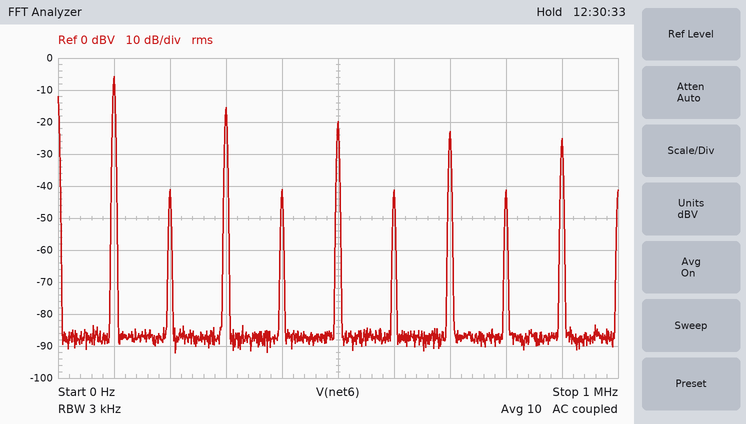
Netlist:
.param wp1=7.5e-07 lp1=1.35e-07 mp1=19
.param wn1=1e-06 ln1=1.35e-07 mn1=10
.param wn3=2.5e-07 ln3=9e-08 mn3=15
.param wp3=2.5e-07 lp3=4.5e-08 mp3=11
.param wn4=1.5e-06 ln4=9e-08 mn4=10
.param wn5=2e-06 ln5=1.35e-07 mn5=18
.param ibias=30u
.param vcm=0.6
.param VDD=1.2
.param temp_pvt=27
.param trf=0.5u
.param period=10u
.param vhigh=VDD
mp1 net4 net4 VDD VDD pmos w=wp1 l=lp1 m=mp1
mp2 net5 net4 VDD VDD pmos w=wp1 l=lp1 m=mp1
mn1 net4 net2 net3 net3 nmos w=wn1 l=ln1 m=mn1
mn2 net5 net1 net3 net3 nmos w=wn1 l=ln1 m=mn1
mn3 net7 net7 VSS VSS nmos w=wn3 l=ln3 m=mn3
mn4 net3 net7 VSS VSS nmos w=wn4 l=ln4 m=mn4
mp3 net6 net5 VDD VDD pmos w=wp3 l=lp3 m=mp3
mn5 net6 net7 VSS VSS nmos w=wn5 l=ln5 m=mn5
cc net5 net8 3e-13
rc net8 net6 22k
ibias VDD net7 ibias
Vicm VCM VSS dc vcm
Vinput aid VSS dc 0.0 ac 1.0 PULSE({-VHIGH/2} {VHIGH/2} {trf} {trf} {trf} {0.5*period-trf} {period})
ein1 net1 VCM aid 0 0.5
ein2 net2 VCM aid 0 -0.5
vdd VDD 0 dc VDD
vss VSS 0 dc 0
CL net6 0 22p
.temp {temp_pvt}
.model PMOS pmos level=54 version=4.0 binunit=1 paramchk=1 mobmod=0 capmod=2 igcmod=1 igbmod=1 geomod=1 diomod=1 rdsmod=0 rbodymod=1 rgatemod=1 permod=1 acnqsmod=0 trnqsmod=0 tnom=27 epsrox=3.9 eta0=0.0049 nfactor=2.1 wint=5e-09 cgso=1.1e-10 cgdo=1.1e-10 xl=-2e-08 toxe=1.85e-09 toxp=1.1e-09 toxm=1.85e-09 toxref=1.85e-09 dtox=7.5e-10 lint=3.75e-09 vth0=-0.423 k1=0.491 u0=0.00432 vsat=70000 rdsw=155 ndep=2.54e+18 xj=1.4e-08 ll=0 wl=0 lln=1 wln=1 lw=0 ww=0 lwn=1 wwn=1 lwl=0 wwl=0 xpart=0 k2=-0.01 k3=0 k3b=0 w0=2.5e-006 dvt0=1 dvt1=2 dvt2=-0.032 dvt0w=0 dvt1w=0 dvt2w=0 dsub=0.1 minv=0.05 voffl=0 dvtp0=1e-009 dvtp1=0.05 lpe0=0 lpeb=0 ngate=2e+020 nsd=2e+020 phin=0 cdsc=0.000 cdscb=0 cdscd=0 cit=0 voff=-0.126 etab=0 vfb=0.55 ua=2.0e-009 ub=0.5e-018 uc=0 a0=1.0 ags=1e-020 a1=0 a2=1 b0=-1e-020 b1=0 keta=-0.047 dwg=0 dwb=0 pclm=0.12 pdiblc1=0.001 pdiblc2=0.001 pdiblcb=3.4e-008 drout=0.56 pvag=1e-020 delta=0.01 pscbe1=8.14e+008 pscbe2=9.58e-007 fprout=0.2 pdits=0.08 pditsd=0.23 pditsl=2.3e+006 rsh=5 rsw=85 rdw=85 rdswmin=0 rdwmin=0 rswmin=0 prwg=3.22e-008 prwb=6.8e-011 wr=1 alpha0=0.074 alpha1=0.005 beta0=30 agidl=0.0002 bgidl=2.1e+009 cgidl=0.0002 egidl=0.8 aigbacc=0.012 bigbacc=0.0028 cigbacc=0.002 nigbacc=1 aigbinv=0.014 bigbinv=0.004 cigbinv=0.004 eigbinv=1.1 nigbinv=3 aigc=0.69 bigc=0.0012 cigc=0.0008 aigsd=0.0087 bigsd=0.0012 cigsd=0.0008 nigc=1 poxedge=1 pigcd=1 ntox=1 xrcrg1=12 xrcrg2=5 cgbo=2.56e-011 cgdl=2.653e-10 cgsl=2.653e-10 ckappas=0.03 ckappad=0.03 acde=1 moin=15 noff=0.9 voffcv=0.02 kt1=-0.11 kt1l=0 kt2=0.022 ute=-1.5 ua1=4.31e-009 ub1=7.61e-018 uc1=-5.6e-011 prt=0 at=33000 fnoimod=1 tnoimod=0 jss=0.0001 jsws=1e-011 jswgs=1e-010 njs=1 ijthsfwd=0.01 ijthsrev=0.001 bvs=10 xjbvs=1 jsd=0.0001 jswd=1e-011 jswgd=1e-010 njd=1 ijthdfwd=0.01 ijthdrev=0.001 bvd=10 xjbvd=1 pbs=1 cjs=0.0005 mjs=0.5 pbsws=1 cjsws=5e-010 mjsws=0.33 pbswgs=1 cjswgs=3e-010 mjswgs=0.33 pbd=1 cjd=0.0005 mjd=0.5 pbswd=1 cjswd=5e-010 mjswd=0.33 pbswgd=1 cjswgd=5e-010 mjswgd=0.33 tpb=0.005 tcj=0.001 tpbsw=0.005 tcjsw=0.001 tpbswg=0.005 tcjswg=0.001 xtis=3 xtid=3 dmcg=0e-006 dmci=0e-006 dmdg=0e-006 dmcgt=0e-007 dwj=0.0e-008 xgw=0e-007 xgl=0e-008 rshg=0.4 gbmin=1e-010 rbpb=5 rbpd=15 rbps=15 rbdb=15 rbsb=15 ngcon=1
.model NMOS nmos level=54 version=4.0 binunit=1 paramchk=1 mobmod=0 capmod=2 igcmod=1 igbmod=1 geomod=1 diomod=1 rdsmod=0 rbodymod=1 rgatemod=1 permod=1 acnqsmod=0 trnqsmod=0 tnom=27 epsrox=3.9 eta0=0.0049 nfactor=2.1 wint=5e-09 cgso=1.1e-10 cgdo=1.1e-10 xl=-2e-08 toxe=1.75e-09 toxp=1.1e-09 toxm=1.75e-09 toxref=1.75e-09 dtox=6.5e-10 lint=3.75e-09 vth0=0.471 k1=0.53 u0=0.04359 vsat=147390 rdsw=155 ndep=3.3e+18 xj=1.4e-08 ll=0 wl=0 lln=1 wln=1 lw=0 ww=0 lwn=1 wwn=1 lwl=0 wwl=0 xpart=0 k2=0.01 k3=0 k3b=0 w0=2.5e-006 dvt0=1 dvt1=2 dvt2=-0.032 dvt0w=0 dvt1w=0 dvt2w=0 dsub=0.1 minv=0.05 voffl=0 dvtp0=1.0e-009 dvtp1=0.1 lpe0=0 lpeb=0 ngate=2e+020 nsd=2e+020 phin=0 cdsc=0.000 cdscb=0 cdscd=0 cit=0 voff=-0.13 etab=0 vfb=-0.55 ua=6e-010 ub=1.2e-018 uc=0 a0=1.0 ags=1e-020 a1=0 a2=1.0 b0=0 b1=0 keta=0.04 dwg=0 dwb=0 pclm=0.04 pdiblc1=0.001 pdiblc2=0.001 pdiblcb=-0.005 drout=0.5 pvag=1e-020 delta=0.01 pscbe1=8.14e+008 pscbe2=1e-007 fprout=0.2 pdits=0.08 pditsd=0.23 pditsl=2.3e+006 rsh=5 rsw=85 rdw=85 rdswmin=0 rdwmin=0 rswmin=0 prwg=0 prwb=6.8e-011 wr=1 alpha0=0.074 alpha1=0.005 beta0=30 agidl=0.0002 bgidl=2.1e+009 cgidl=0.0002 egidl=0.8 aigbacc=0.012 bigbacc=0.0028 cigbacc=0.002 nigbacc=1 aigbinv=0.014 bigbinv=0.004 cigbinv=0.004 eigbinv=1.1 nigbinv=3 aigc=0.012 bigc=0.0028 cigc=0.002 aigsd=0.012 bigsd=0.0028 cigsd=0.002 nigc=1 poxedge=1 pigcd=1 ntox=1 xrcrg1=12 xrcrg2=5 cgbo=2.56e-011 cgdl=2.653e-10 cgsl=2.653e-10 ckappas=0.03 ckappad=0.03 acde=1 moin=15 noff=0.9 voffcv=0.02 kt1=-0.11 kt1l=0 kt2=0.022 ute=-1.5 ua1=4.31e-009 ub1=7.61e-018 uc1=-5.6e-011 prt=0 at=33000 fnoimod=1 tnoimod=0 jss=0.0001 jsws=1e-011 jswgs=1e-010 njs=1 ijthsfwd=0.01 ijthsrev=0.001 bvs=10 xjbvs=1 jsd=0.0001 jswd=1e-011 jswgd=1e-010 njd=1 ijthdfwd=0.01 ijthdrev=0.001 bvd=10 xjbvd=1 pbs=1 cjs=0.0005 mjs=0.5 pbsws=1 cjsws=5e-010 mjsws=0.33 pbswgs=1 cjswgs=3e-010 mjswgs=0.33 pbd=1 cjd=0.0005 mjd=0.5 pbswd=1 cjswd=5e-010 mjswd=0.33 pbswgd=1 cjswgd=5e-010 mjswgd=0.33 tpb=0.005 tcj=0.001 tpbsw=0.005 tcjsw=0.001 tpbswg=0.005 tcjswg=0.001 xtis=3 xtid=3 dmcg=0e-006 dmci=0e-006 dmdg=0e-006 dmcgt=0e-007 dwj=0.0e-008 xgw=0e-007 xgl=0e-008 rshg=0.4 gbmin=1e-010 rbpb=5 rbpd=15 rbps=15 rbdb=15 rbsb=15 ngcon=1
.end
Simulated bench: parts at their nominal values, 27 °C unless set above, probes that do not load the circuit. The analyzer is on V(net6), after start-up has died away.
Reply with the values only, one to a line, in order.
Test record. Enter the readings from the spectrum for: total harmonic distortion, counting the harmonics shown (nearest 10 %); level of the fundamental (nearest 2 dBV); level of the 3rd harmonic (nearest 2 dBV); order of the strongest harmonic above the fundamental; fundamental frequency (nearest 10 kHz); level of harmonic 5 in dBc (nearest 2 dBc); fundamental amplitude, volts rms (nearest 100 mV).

40 %
-6 dBV
-16 dBV
3
100 kHz
-14 dBc
500 mV
